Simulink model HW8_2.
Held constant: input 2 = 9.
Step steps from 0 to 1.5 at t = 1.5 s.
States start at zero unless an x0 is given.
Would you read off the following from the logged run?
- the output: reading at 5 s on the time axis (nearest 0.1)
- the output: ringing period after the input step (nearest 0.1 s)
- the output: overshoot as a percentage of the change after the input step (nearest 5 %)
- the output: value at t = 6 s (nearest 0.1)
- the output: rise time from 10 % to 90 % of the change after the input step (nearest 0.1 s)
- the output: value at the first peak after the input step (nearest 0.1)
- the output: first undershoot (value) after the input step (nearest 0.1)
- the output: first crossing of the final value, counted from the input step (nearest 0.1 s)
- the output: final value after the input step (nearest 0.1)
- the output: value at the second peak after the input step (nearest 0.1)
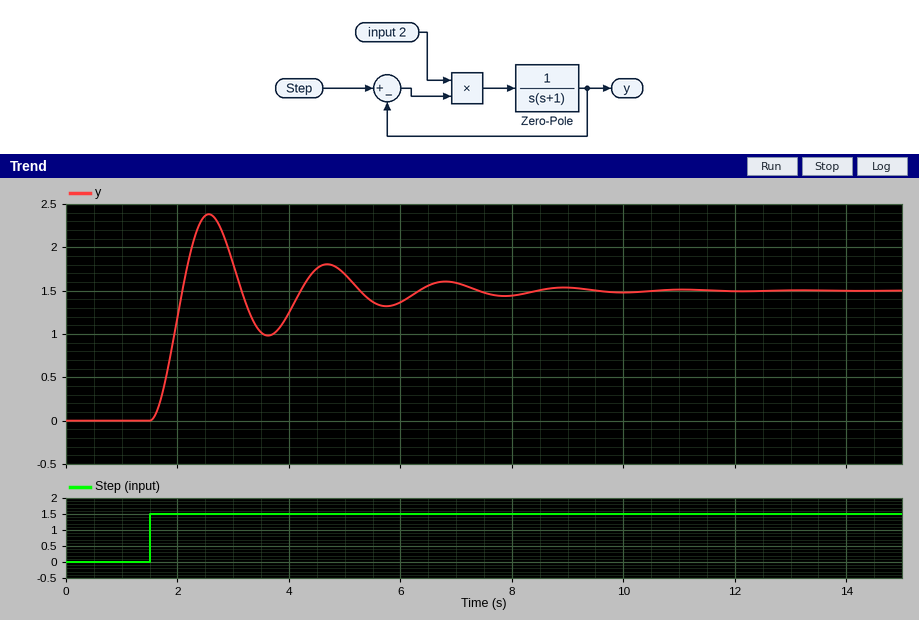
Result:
1.7
2.1 s
60 %
1.4
0.4 s
2.4
1.0
0.6 s
1.5
1.8
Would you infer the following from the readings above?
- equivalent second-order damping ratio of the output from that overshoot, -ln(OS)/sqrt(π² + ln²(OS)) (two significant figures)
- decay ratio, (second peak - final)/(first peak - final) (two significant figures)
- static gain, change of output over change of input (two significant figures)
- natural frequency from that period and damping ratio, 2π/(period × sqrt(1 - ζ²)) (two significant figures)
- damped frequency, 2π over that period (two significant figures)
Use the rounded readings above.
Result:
0.16
0.33
1.0
3.0 rad/s
3.0 rad/s
